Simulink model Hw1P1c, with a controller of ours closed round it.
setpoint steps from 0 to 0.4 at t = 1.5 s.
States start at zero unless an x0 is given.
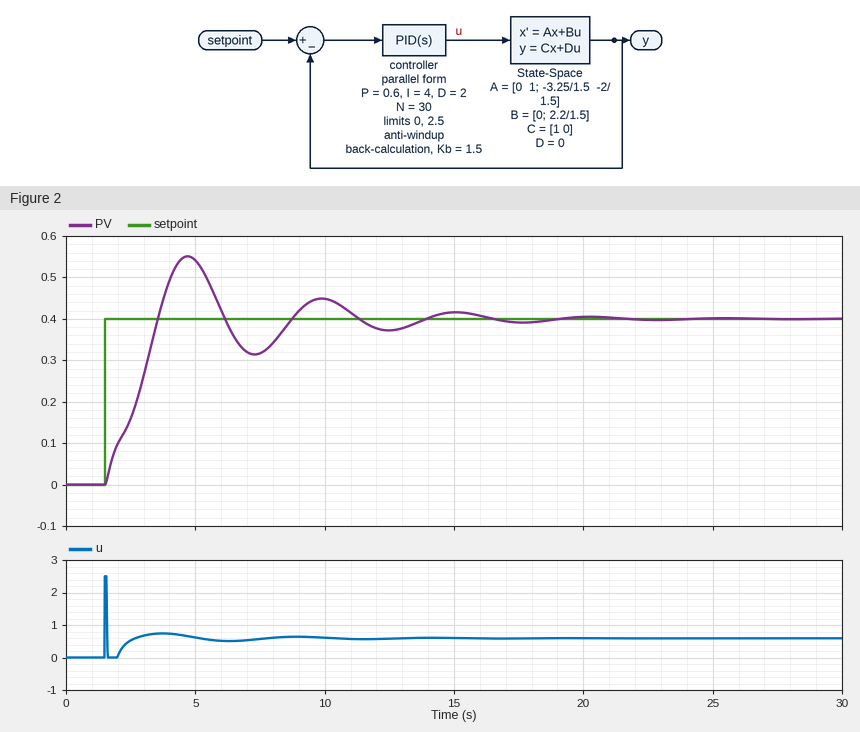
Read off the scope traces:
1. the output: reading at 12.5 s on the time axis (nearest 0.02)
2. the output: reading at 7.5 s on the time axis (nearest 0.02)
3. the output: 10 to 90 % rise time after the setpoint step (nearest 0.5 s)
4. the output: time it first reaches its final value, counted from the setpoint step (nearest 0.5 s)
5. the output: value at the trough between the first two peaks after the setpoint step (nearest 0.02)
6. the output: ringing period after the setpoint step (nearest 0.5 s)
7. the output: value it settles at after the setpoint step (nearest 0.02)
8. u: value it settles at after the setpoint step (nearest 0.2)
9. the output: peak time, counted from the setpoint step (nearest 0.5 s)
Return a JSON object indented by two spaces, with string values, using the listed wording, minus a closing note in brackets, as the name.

{
  "the output: reading at 12.5 s on the time axis": "0.38",
  "the output: reading at 7.5 s on the time axis": "0.32",
  "the output: 10 to 90 % rise time after the setpoint step": "1.5 s",
  "the output: time it first reaches its final value, counted from the setpoint step": "2.0 s",
  "the output: value at the trough between the first two peaks after the setpoint step": "0.32",
  "the output: ringing period after the setpoint step": "5.0 s",
  "the output: value it settles at after the setpoint step": "0.40",
  "u: value it settles at after the setpoint step": "0.6",
  "the output: peak time, counted from the setpoint step": "3.0 s"
}
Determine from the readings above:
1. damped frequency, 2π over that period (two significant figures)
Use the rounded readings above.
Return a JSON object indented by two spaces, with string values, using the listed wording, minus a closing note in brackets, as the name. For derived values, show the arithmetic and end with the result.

{
  "damped frequency, 2π over that period": "2π / 5 = 1.3 rad/s"
}
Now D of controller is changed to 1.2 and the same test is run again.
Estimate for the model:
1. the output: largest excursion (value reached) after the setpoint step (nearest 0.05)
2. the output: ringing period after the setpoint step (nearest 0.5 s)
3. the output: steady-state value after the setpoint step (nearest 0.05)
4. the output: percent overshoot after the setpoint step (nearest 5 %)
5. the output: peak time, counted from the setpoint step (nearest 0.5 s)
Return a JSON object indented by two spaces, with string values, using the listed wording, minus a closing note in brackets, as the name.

{
  "the output: largest excursion (value reached) after the setpoint step": "0.55",
  "the output: ringing period after the setpoint step": "4.5 s",
  "the output: steady-state value after the setpoint step": "0.40",
  "the output: percent overshoot after the setpoint step": "40 %",
  "the output: peak time, counted from the setpoint step": "2.5 s"
}
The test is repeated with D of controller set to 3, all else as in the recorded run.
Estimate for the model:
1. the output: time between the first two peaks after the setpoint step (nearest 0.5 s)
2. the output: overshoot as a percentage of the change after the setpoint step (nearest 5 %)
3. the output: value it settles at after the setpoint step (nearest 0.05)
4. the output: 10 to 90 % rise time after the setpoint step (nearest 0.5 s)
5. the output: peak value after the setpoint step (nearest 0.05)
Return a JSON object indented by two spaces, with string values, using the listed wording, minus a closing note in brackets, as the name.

{
  "the output: time between the first two peaks after the setpoint step": "6.0 s",
  "the output: overshoot as a percentage of the change after the setpoint step": "35 %",
  "the output: value it settles at after the setpoint step": "0.40",
  "the output: 10 to 90 % rise time after the setpoint step": "2.0 s",
  "the output: peak value after the setpoint step": "0.55"
}
